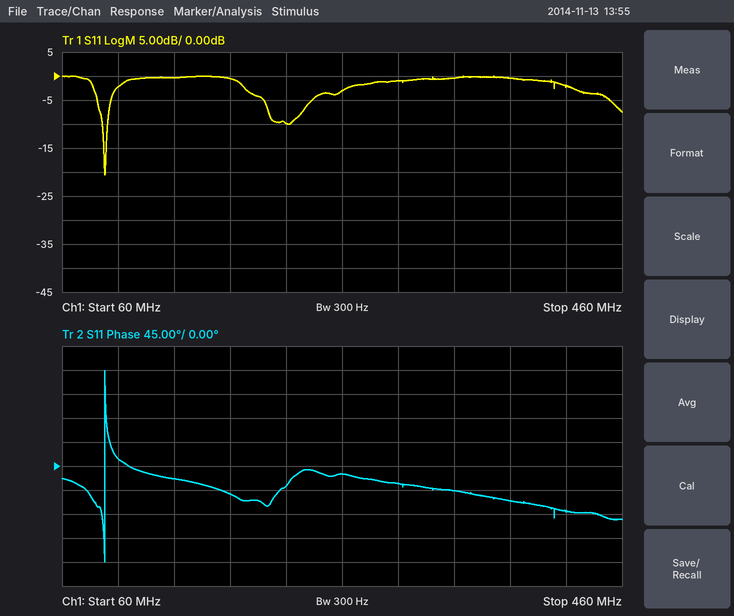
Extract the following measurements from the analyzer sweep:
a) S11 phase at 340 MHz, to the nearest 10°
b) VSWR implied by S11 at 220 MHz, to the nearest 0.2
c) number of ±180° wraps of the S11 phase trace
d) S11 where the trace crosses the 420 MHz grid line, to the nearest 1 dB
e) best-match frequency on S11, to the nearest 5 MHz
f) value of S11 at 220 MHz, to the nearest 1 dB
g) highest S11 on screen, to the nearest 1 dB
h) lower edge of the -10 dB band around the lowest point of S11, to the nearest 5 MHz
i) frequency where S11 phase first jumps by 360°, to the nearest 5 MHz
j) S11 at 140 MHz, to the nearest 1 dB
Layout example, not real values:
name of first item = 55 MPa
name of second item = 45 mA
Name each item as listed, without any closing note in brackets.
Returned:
S11 phase at 340 MHz, to the nearest 10° = -50°
VSWR implied by S11 at 220 MHz, to the nearest 0.2 = 2.0
number of ±180° wraps of the S11 phase trace = 1
S11 where the trace crosses the 420 MHz grid line, to the nearest 1 dB = -2 dB
best-match frequency on S11, to the nearest 5 MHz = 90 MHz
value of S11 at 220 MHz, to the nearest 1 dB = -10 dB
highest S11 on screen, to the nearest 1 dB = 0 dB
lower edge of the -10 dB band around the lowest point of S11, to the nearest 5 MHz = 90 MHz
frequency where S11 phase first jumps by 360°, to the nearest 5 MHz = 90 MHz
S11 at 140 MHz, to the nearest 1 dB = 0 dB
